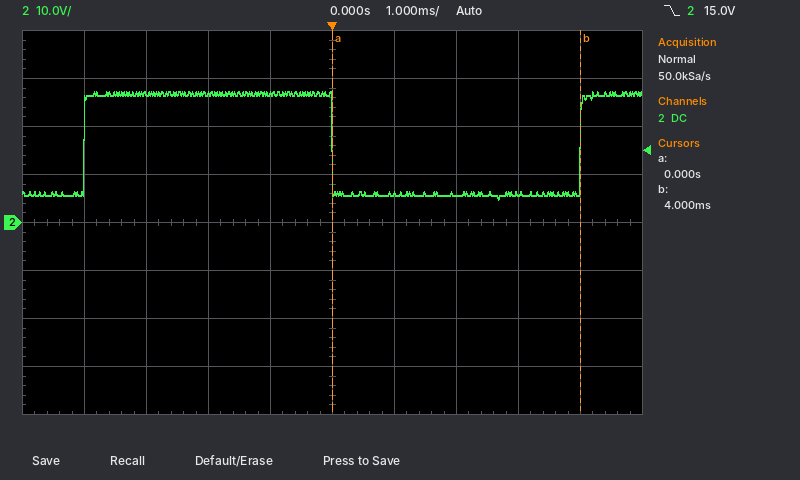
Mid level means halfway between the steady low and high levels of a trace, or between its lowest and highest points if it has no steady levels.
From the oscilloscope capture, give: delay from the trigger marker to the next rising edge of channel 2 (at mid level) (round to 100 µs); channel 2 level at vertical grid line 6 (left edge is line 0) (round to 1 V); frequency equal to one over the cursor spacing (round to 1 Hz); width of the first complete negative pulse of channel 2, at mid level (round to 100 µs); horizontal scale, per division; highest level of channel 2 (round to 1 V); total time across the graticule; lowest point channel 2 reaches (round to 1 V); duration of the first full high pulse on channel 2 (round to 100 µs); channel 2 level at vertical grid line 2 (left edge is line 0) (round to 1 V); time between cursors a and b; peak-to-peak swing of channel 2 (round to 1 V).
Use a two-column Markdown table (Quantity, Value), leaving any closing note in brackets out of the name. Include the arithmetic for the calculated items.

| Quantity | Value |
|---|---|
| delay from the trigger marker to the next rising edge of channel 2 (at mid level) | 4.0 ms |
| channel 2 level at vertical grid line 6 (left edge is line 0) | 6 V |
| frequency equal to one over the cursor spacing | 1 / 4.0 ms ≈ 250 Hz |
| width of the first complete negative pulse of channel 2, at mid level | 4.0 ms |
| horizontal scale, per division | 1 ms |
| highest level of channel 2 | 27 V |
| total time across the graticule | 10 ms |
| lowest point channel 2 reaches | 5 V |
| duration of the first full high pulse on channel 2 | 4.0 ms |
| channel 2 level at vertical grid line 2 (left edge is line 0) | 27 V |
| time between cursors a and b | 4 ms − (0 s) = 4.0 ms |
| peak-to-peak swing of channel 2 | 27 V − (5 V) = 22 V |
